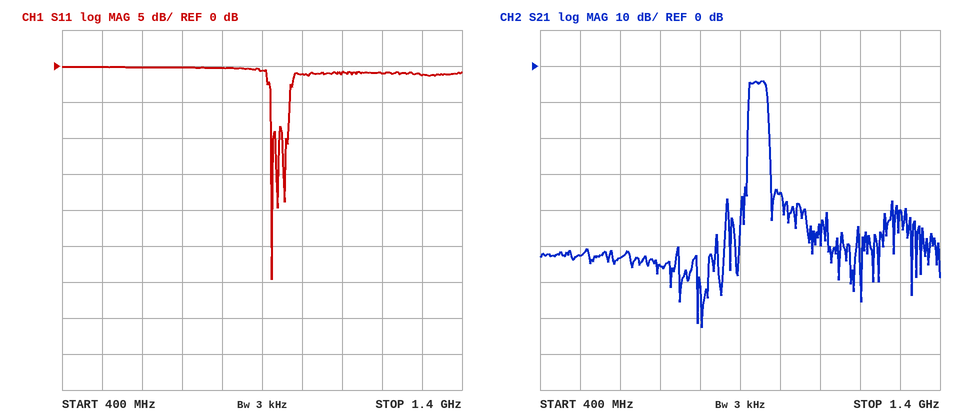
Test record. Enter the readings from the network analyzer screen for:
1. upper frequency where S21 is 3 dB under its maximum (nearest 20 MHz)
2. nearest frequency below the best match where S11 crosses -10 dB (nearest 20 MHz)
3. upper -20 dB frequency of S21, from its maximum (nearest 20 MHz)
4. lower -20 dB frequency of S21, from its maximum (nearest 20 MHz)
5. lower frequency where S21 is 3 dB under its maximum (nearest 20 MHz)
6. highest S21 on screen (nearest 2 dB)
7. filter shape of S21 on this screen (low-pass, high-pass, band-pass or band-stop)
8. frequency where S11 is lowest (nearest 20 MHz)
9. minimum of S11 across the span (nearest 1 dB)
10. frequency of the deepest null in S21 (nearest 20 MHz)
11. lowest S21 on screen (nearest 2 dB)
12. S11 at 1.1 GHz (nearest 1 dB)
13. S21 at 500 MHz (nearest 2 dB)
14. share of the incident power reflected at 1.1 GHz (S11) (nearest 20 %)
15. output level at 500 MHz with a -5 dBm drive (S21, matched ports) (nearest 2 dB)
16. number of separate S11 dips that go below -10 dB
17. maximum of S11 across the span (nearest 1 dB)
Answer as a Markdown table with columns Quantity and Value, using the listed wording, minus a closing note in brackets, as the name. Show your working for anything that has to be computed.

| Quantity | Value |
|---|---|
| upper frequency where S21 is 3 dB under its maximum | 960 MHz |
| nearest frequency below the best match where S11 crosses -10 dB | 920 MHz |
| upper -20 dB frequency of S21, from its maximum | 980 MHz |
| lower -20 dB frequency of S21, from its maximum | 920 MHz |
| lower frequency where S21 is 3 dB under its maximum | 920 MHz |
| highest S21 on screen | -4 dB |
| filter shape of S21 on this screen | band-pass |
| frequency where S11 is lowest | 920 MHz |
| minimum of S11 across the span | -30 dB |
| frequency of the deepest null in S21 | 800 MHz |
| lowest S21 on screen | -72 dB |
| S11 at 1.1 GHz | -1 dB |
| S21 at 500 MHz | -52 dB |
| share of the incident power reflected at 1.1 GHz (S11) | 10^(-1/10) ≈ 79.4 %, so 80 % to the nearest 20 % |
| output level at 500 MHz with a -5 dBm drive (S21, matched ports) | -5 dBm + (-52 dB) = -58 dBm |
| number of separate S11 dips that go below -10 dB | 3 |
| maximum of S11 across the span | 0 dB |
